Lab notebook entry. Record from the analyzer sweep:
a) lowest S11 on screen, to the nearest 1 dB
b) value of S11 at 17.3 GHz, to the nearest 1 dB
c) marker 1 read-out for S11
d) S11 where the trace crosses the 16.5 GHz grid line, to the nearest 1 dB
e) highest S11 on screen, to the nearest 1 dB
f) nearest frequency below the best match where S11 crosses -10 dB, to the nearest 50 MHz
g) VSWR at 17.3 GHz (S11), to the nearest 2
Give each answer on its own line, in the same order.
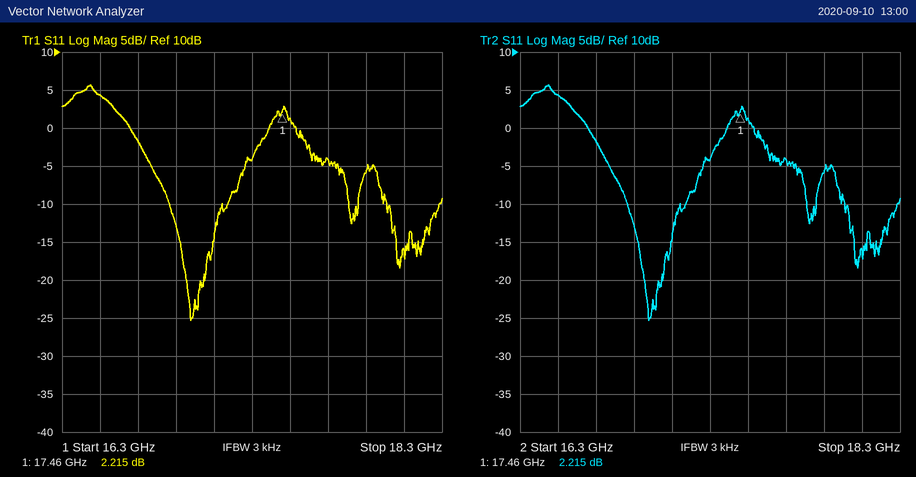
-25 dB
-4 dB
2.215 dB
4 dB
6 dB
16.85 GHz
4
